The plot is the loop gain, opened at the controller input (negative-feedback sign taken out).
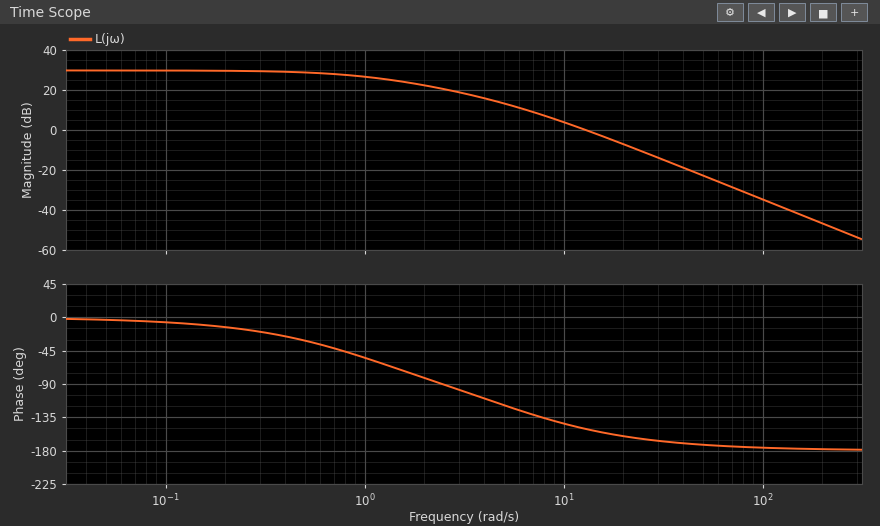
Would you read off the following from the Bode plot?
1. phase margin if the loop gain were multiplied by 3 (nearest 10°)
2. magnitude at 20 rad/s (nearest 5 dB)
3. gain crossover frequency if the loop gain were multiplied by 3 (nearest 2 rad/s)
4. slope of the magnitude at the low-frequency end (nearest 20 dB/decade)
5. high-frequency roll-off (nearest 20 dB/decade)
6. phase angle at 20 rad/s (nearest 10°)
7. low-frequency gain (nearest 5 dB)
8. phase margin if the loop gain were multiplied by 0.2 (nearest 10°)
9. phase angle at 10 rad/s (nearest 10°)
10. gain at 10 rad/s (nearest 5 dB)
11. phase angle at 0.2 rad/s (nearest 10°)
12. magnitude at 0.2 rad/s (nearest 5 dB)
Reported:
20°
-5 dB
24 rad/s
0 dB/decade
-40 dB/decade
-160°
30 dB
60°
-140°
5 dB
-10°
30 dB
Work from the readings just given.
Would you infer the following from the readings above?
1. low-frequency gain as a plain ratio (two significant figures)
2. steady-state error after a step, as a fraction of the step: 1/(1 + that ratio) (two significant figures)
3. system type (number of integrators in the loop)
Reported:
32
0.030
0
